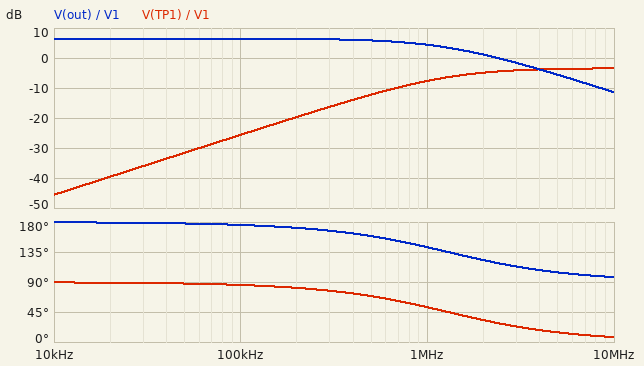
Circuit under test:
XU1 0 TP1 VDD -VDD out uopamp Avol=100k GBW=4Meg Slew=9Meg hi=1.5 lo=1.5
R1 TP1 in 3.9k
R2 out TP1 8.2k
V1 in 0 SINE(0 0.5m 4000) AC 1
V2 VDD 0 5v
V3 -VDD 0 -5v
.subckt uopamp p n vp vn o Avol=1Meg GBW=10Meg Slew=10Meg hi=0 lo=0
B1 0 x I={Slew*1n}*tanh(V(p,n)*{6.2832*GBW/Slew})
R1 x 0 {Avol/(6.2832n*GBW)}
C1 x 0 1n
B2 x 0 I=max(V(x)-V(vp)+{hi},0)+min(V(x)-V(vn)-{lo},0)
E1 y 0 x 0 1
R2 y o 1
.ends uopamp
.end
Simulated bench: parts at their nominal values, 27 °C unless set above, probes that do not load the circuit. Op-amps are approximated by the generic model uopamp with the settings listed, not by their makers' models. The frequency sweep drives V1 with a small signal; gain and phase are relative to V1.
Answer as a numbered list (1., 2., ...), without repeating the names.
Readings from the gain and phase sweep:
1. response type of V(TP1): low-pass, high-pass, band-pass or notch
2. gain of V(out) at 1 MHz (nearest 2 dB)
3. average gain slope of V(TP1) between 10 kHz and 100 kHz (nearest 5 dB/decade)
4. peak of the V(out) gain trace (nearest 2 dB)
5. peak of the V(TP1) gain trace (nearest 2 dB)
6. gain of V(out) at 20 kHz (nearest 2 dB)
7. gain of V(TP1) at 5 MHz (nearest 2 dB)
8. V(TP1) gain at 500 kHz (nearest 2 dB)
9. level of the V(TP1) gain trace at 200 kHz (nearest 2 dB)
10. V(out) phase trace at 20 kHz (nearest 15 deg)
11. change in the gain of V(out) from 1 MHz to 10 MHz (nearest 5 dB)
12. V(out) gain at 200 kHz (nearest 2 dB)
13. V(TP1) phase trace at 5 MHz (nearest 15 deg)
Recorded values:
1. high-pass
2. 4 dB
3. 20 dB/decade
4. 6 dB
5. -4 dB
6. 6 dB
7. -4 dB
8. -12 dB
9. -20 dB
10. 180 deg
11. -15 dB
12. 6 dB
13. 15 deg
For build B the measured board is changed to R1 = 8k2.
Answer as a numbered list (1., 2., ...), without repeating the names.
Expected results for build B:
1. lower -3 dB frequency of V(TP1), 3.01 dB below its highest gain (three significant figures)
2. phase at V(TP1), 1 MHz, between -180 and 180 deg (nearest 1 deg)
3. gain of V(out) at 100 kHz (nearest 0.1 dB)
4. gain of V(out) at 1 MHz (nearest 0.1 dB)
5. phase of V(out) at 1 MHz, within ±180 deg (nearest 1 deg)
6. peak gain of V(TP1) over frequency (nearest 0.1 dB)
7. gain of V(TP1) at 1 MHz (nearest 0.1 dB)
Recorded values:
1. 2.00 MHz
2. 63 deg
3. 0 dB
4. -1.0 dB
5. 153 deg
6. -6.0 dB
7. -13.0 dB
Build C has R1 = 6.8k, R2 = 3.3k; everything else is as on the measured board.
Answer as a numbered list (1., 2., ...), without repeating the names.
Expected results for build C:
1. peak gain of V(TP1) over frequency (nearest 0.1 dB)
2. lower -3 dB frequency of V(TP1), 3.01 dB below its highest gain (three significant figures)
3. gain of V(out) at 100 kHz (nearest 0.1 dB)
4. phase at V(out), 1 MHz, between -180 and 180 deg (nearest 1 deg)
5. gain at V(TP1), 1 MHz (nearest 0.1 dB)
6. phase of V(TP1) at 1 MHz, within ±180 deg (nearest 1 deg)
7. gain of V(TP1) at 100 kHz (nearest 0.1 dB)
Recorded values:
1. -9.7 dB
2. 2.69 MHz
3. -6.3 dB
4. 160 deg
5. -18.9 dB
6. 70 deg
7. -38.3 dB
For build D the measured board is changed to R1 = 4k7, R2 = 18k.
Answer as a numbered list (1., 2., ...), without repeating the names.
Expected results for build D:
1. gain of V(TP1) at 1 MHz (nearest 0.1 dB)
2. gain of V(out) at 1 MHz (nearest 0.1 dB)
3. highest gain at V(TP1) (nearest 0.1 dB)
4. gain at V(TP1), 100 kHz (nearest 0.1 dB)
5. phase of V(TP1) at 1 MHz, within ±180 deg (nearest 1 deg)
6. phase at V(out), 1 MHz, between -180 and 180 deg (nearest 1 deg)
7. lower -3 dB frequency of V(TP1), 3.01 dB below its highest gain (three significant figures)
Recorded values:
1. -4.3 dB
2. 7.8 dB
3. -2.0 dB
4. -20.4 dB
5. 40 deg
6. 130 deg
7. 828 kHz
